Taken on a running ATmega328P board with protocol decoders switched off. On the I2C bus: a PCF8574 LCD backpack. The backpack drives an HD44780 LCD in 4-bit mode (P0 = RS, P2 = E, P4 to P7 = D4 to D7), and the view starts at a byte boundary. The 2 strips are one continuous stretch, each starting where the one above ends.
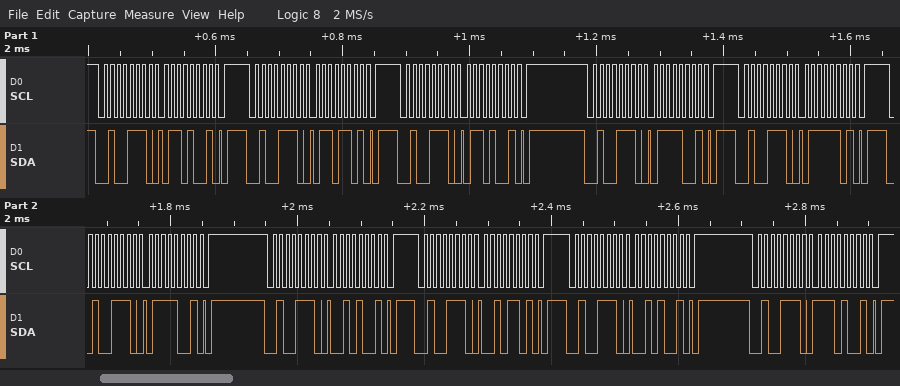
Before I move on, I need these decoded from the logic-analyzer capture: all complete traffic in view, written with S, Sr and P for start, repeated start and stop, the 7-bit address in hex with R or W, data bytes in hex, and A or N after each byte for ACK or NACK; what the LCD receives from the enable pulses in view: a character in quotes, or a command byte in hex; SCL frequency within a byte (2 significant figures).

S 27W A 69 A P S 27W A 6D A P S 27W A 69 A P S 27W A 79 A P S 27W A 7D A P S 27W A 79 A P S 27W A 29 A P S 27W A 2D A P S 27W A 29 A P S 27W A E9 A P
'g'
100 kHz
